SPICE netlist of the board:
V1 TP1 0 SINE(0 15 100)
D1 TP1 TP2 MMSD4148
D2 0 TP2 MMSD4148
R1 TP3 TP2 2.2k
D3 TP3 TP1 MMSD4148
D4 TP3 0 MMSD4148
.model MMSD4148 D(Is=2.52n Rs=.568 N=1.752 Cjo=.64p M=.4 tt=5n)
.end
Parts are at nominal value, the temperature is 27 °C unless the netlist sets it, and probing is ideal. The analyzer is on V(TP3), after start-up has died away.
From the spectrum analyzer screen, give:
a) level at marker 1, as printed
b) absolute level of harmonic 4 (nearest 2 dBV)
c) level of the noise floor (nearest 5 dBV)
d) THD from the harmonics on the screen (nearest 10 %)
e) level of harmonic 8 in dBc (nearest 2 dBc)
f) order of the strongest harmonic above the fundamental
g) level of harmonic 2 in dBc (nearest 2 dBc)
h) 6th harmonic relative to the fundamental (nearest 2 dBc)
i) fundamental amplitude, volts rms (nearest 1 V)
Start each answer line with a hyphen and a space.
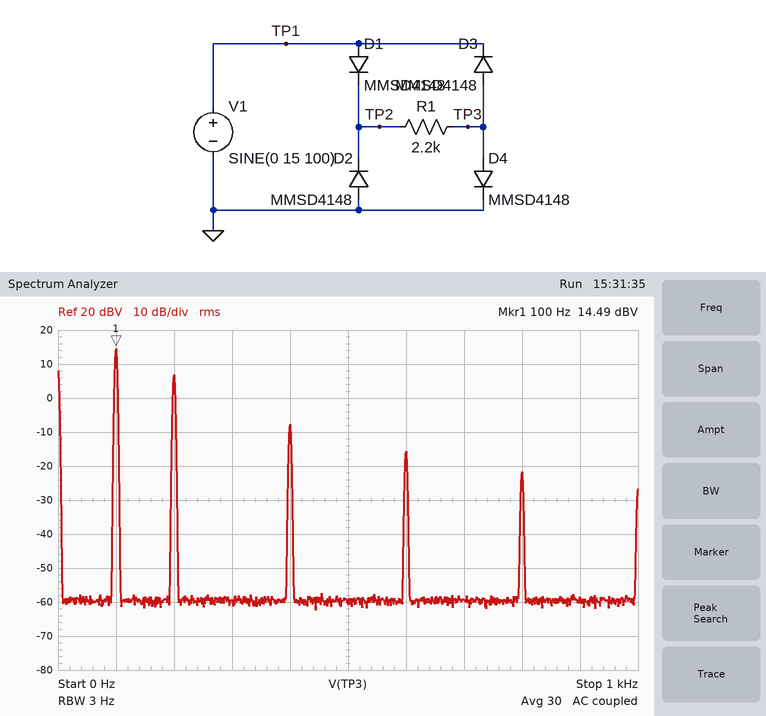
- 14.49 dBV
- -8 dBV
- -60 dBV
- 40 %
- -36 dBc
- 2
- -8 dBc
- -30 dBc
- 5 V
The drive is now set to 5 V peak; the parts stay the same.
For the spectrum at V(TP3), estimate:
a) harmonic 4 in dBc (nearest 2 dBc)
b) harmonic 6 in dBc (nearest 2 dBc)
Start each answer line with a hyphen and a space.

- -26 dBc
- -40 dBc
